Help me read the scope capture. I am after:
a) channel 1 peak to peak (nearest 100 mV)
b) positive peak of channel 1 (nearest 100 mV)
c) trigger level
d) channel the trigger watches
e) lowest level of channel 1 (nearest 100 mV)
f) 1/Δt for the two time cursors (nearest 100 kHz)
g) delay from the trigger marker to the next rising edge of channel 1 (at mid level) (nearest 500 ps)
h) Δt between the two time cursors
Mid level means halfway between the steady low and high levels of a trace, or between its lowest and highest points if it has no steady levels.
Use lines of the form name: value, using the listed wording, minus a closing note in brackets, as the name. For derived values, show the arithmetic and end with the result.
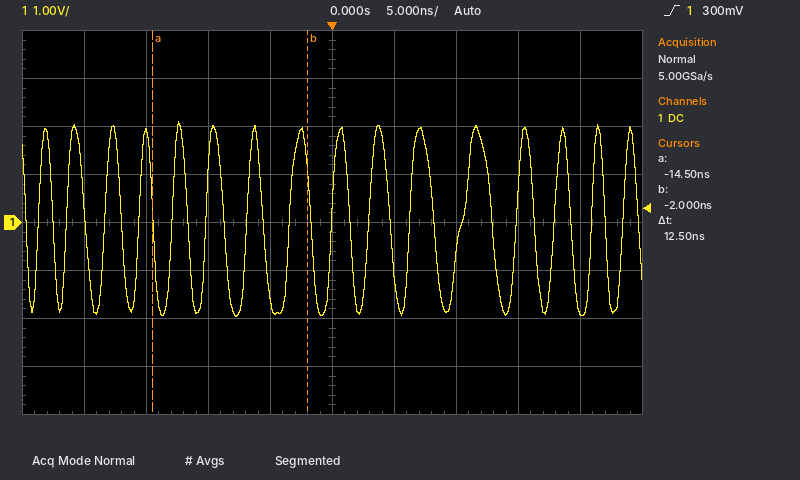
channel 1 peak to peak: 2.1 V − (-2.0 V) = 4.1 V
positive peak of channel 1: 2.1 V
trigger level: 300 mV
channel the trigger watches: channel 1
lowest level of channel 1: -2.0 V
1/Δt for the two time cursors: 1 / 12.5 ns ≈ 80.0 MHz
delay from the trigger marker to the next rising edge of channel 1 (at mid level): 3.0 ns
Δt between the two time cursors: 12.5 ns
